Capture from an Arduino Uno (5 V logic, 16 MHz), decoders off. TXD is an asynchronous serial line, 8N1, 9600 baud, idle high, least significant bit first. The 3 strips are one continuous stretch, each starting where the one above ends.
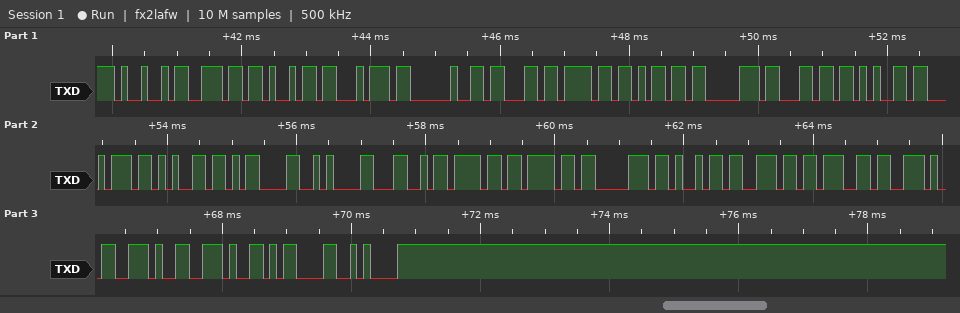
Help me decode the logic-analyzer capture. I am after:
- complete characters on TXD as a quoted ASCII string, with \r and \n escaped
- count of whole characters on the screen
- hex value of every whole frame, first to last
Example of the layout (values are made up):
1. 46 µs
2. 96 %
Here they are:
1. "Init complete\r\nLooping...\r\n"
2. 27
3. 0x49 0x6E 0x69 0x74 0x20 0x63 0x6F 0x6D 0x70 0x6C 0x65 0x74 0x65 0x0D 0x0A 0x4C 0x6F 0x6F 0x70 0x69 0x6E 0x67 0x2E 0x2E 0x2E 0x0D 0x0A
